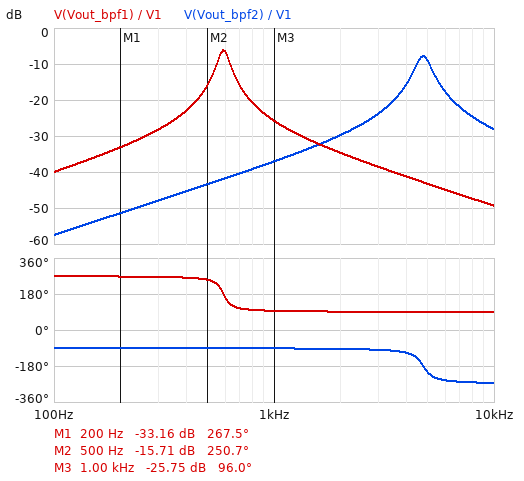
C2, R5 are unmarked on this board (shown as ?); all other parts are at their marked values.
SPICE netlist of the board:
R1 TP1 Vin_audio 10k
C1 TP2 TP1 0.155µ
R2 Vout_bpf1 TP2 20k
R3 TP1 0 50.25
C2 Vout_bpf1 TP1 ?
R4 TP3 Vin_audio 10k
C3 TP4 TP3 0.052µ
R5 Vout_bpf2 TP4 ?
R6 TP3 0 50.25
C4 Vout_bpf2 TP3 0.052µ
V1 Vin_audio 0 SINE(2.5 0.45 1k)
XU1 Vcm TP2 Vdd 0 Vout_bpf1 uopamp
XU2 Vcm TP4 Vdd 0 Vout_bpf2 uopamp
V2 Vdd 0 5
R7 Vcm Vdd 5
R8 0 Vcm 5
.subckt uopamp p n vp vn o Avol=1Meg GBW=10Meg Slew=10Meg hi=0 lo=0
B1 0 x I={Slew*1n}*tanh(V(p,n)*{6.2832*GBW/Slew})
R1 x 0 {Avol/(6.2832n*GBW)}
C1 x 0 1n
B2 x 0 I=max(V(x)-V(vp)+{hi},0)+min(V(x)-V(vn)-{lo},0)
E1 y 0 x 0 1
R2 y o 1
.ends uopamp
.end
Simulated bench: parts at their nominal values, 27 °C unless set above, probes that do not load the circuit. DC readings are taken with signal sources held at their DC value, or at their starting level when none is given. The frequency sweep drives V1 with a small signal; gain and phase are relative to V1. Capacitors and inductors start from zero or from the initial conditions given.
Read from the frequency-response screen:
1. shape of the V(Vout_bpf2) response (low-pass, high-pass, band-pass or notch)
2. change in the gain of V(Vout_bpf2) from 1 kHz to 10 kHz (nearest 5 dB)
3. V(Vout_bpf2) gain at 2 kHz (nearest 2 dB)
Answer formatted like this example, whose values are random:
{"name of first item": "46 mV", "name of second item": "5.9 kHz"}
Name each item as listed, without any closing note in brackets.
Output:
{"shape of the V(Vout_bpf2) response": "band-pass", "change in the gain of V(Vout_bpf2) from 1 kHz to 10 kHz": "10 dB", "V(Vout_bpf2) gain at 2 kHz": "-30 dB"}
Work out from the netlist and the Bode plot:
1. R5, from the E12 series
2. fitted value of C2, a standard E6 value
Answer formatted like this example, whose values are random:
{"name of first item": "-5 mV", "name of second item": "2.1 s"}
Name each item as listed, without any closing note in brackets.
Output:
{"R5, from the E12 series": "8.2 kΩ", "fitted value of C2, a standard E6 value": "470 nF"}
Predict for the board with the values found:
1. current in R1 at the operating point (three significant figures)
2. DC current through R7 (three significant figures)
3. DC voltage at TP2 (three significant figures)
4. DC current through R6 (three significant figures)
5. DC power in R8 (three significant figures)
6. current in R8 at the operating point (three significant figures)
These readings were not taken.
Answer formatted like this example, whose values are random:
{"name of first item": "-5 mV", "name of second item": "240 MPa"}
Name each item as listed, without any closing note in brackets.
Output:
{"current in R1 at the operating point": "249 µA", "DC current through R7": "500 mA", "DC voltage at TP2": "2.50 V", "DC current through R6": "249 µA", "DC power in R8": "1.25 W", "current in R8 at the operating point": "500 mA"}
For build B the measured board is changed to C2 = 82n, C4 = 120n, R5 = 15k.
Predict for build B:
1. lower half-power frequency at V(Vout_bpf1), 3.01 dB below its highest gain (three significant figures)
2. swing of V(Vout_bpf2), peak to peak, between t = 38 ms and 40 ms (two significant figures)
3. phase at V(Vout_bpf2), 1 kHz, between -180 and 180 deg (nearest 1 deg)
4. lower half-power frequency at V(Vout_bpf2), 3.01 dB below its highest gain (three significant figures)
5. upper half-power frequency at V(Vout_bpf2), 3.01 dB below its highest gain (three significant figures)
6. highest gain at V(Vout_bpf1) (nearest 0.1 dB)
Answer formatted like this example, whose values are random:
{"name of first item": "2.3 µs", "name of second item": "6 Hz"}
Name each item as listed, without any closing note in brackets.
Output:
{"lower half-power frequency at V(Vout_bpf1), 3.01 dB below its highest gain": "1.34 kHz", "swing of V(Vout_bpf2), peak to peak, between t = 38 ms and 40 ms": "27 mV", "phase at V(Vout_bpf2), 1 kHz, between -180 and 180 deg": "-94 deg", "lower half-power frequency at V(Vout_bpf2), 3.01 dB below its highest gain": "2.18 kHz", "upper half-power frequency at V(Vout_bpf2), 3.01 dB below its highest gain": "2.47 kHz", "highest gain at V(Vout_bpf1)": "2.3 dB"}
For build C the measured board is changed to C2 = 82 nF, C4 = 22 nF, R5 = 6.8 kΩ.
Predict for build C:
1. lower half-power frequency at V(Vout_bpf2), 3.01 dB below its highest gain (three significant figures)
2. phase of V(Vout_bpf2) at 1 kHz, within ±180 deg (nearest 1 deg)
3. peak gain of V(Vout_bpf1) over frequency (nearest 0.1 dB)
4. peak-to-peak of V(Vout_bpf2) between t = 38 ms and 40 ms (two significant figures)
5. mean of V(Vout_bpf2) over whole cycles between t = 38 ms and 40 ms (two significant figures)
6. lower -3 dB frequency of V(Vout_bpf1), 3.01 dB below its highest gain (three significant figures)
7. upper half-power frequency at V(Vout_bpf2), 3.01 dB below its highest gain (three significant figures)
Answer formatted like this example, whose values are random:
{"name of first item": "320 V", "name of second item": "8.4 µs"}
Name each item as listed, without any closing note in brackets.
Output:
{"lower half-power frequency at V(Vout_bpf2), 3.01 dB below its highest gain": "7.30 kHz", "phase of V(Vout_bpf2) at 1 kHz, within ±180 deg": "-91 deg", "peak gain of V(Vout_bpf1) over frequency": "2.3 dB", "peak-to-peak of V(Vout_bpf2) between t = 38 ms and 40 ms": "10 mV", "mean of V(Vout_bpf2) over whole cycles between t = 38 ms and 40 ms": "2.5 V", "lower -3 dB frequency of V(Vout_bpf1), 3.01 dB below its highest gain": "1.34 kHz", "upper half-power frequency at V(Vout_bpf2), 3.01 dB below its highest gain": "8.79 kHz"}
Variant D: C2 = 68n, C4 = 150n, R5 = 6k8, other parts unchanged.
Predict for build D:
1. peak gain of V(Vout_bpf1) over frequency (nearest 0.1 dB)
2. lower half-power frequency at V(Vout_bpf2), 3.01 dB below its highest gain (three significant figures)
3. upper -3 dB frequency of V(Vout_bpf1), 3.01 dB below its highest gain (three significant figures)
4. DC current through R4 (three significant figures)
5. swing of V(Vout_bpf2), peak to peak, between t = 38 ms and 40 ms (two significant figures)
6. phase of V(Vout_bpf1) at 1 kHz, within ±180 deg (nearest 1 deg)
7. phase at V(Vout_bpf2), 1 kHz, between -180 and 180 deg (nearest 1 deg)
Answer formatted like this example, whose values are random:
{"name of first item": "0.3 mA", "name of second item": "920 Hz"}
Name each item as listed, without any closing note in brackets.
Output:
{"peak gain of V(Vout_bpf1) over frequency": "2.9 dB", "lower half-power frequency at V(Vout_bpf2), 3.01 dB below its highest gain": "2.80 kHz", "upper -3 dB frequency of V(Vout_bpf1), 3.01 dB below its highest gain": "1.63 kHz", "DC current through R4": "249 µA", "swing of V(Vout_bpf2), peak to peak, between t = 38 ms and 40 ms": "11 mV", "phase of V(Vout_bpf1) at 1 kHz, within ±180 deg": "-97 deg", "phase at V(Vout_bpf2), 1 kHz, between -180 and 180 deg": "-94 deg"}
